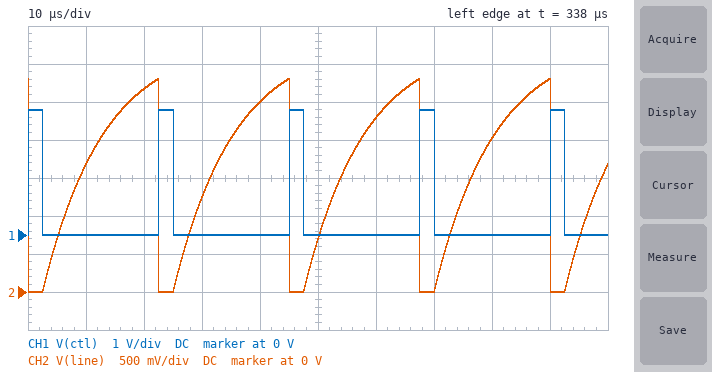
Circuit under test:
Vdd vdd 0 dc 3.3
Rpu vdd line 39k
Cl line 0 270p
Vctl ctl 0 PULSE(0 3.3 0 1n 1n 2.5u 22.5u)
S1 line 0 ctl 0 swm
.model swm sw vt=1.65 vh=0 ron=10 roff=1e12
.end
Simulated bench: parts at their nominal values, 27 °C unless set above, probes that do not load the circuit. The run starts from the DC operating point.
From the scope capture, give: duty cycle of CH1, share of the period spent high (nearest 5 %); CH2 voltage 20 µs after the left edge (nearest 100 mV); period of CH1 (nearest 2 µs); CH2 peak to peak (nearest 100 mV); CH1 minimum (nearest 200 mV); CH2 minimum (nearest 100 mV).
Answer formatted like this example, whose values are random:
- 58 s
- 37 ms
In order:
- 10 %
- 2.7 V
- 22 µs
- 2.8 V
- 0 V
- 0 V
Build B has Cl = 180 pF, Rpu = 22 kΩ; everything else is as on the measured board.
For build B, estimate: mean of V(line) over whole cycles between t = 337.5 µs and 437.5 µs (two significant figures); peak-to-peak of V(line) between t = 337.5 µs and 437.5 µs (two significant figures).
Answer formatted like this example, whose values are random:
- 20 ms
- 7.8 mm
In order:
- 2.4 V
- 3.3 V
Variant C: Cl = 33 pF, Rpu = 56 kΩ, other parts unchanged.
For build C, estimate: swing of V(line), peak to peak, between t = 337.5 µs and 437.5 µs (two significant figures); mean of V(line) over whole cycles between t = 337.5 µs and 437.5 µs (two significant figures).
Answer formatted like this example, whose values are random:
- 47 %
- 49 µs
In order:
- 3.3 V
- 2.7 V
